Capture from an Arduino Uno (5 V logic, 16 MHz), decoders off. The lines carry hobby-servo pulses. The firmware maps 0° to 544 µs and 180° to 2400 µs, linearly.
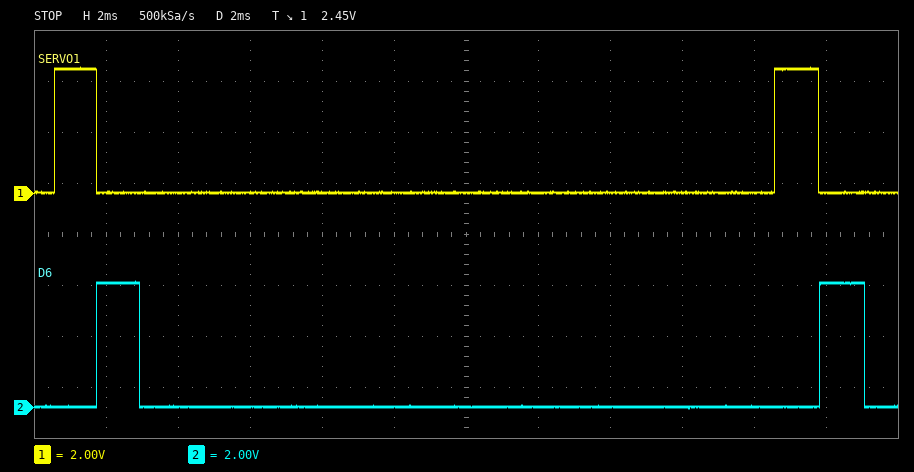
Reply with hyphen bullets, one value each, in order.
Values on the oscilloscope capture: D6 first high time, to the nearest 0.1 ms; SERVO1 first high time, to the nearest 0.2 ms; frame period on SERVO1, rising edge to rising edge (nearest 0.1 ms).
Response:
- 1.2 ms
- 1.2 ms
- 20.0 ms
